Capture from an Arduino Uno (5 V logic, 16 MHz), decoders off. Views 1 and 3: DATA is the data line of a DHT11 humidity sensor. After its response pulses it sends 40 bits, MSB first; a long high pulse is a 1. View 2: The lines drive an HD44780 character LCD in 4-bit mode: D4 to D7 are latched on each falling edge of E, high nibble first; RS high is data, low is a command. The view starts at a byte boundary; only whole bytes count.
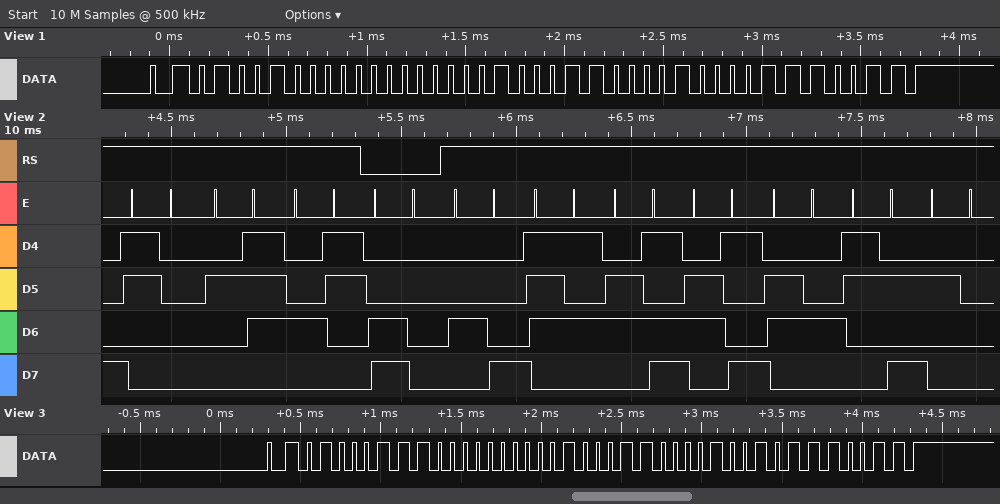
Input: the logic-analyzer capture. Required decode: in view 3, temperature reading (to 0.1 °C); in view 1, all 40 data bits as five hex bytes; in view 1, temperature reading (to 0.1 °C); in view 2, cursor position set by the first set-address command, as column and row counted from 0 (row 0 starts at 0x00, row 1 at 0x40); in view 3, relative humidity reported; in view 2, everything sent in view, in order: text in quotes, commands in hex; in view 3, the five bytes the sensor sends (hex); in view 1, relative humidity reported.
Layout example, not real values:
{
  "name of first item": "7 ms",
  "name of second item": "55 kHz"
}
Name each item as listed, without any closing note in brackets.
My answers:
{
  "in view 3, temperature reading": "35.9 °C",
  "in view 1, all 40 data bits as five hex bytes": "48 00 23 08 73",
  "in view 1, temperature reading": "35.8 °C",
  "in view 2, cursor position set by the first set-address command, as column and row counted from 0": "column 0, row 1",
  "in view 3, relative humidity reported": "71 %",
  "in view 2, everything sent in view, in order: text in quotes, commands in hex": "\"0'C\" 0xC0 \"Humid: \"",
  "in view 3, the five bytes the sensor sends": "47 00 23 09 73",
  "in view 1, relative humidity reported": "72 %"
}
